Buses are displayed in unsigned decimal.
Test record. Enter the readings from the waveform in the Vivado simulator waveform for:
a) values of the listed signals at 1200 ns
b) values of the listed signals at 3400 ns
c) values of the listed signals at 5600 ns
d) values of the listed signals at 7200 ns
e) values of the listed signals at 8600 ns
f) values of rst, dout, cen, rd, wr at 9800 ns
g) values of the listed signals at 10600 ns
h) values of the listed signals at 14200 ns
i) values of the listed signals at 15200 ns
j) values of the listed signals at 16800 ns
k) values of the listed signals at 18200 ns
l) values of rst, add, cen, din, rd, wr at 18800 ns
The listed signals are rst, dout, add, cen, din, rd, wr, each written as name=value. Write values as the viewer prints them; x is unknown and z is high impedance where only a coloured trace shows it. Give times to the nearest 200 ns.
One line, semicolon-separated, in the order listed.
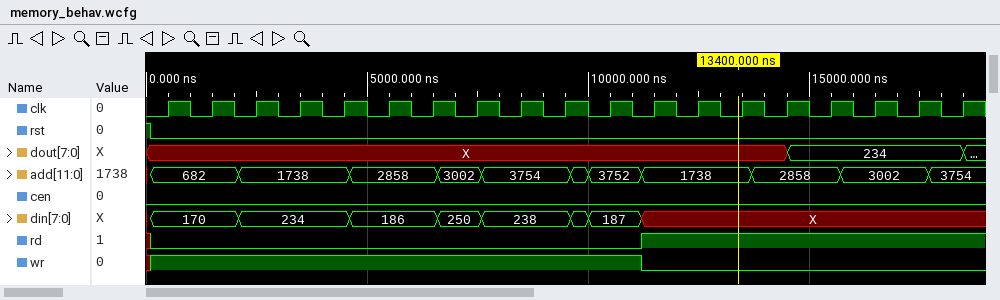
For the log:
rst=0, dout=X, add=682, cen=0, din=170, rd=0, wr=1; rst=0, dout=X, add=1738, cen=0, din=234, rd=0, wr=1; rst=0, dout=X, add=2858, cen=0, din=186, rd=0, wr=1; rst=0, dout=X, add=3002, cen=0, din=250, rd=0, wr=1; rst=0, dout=X, add=3754, cen=0, din=238, rd=0, wr=1; rst=0, dout=X, cen=0, rd=0, wr=1; rst=0, dout=X, add=3752, cen=0, din=187, rd=0, wr=1; rst=0, dout=X, add=2858, cen=0, din=X, rd=1, wr=0; rst=0, dout=234, add=2858, cen=0, din=X, rd=1, wr=0; rst=0, dout=234, add=3002, cen=0, din=X, rd=1, wr=0; rst=0, dout=234, add=3754, cen=0, din=X, rd=1, wr=0; rst=0, add=3754, cen=0, din=X, rd=1, wr=0
